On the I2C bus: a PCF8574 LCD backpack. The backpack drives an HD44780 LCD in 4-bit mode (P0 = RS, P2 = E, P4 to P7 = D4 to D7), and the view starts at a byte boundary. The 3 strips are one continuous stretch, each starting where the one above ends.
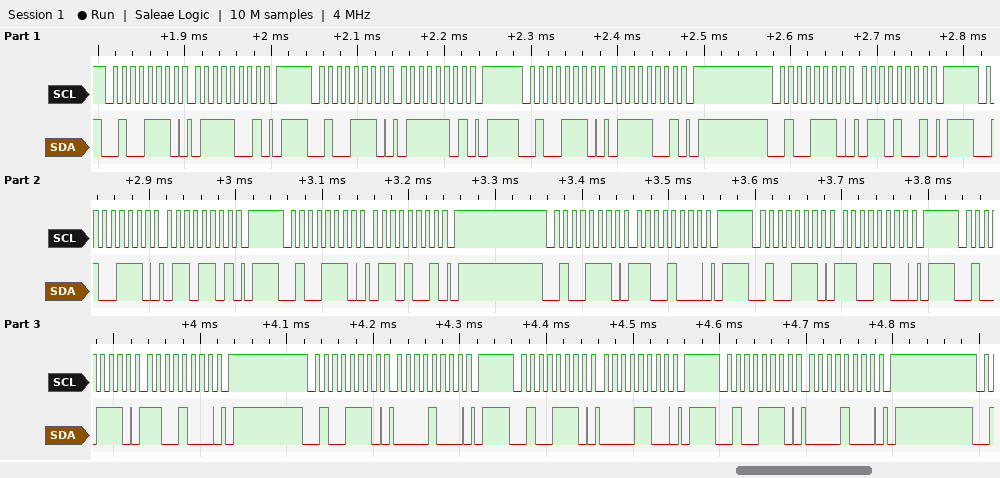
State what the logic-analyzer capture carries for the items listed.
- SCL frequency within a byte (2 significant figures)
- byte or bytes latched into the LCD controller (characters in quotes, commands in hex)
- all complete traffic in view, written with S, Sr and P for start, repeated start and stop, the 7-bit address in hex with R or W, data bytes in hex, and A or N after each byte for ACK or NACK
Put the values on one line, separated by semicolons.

100 kHz; 'v' 0xC0; S 27W A 79 A P S 27W A 7D A P S 27W A 79 A P S 27W A 69 A P S 27W A 6D A P S 27W A 69 A P S 27W A C8 A P S 27W A CC A P S 27W A C8 A P S 27W A 08 A P S 27W A 0C A P S 27W A 08 A P
